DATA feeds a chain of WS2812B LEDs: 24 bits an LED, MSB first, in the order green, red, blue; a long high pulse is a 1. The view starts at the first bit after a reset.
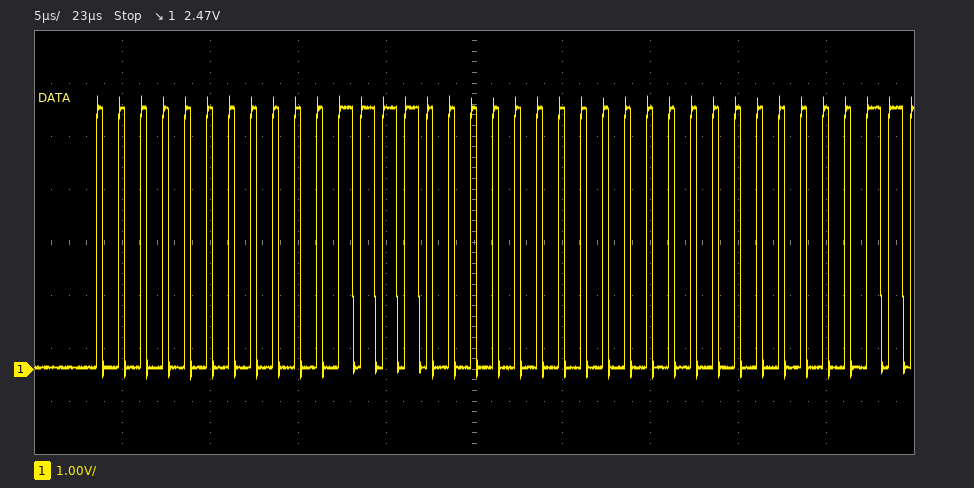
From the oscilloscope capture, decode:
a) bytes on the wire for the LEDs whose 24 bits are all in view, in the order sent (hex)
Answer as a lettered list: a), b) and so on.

a) 00 1E 00
